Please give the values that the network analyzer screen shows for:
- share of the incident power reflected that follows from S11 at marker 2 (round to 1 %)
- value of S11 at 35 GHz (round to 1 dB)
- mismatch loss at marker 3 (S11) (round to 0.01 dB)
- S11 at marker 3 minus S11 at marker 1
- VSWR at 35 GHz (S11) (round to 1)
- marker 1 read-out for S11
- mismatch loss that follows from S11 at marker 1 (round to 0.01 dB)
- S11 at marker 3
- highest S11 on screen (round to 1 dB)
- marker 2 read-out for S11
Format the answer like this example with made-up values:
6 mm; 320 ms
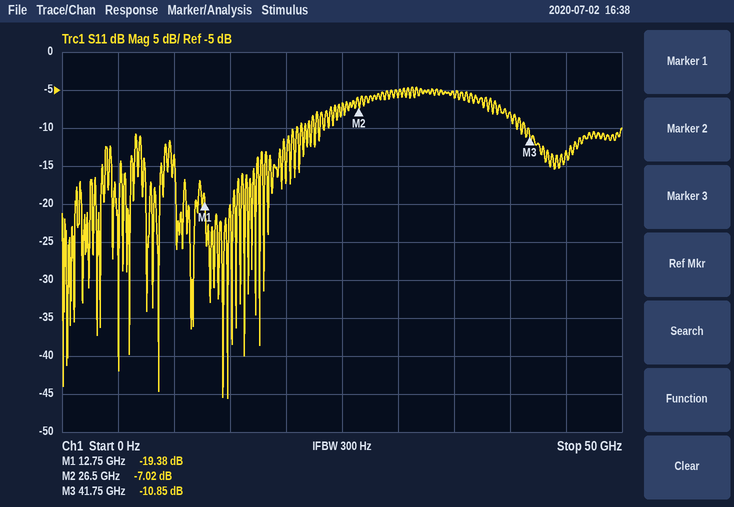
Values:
20 %; -6 dB; 0.37 dB; 8.53 dB; 3; -19.38 dB; 0.05 dB; -10.85 dB; -5 dB; -7.02 dB
